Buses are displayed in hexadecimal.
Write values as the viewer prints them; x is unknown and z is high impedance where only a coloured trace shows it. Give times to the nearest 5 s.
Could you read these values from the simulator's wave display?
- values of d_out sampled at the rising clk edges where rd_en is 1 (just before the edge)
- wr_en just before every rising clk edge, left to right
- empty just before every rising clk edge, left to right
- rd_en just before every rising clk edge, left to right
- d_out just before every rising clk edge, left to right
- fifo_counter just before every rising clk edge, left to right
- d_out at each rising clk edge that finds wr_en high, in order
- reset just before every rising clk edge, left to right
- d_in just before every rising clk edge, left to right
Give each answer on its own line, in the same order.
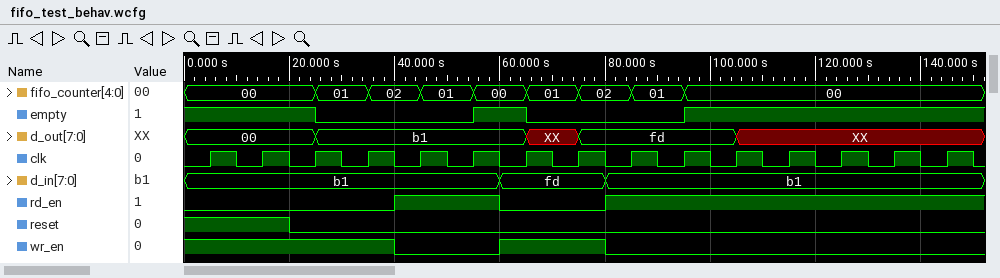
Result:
b1, b1, fd, fd, fd, XX, XX, XX, XX
1 1 1 1 0 0 1 1 0 0 0 0 0 0 0
1 1 1 0 0 0 1 0 0 0 1 1 1 1 1
0 0 0 0 1 1 0 0 1 1 1 1 1 1 1
00, 00, 00, b1, b1, b1, b1, XX, fd, fd, fd, XX, XX, XX, XX
00, 00, 00, 01, 02, 01, 00, 01, 02, 01, 00, 00, 00, 00, 00
00, 00, 00, b1, b1, XX
1 1 0 0 0 0 0 0 0 0 0 0 0 0 0
b1, b1, b1, b1, b1, b1, fd, fd, b1, b1, b1, b1, b1, b1, b1
